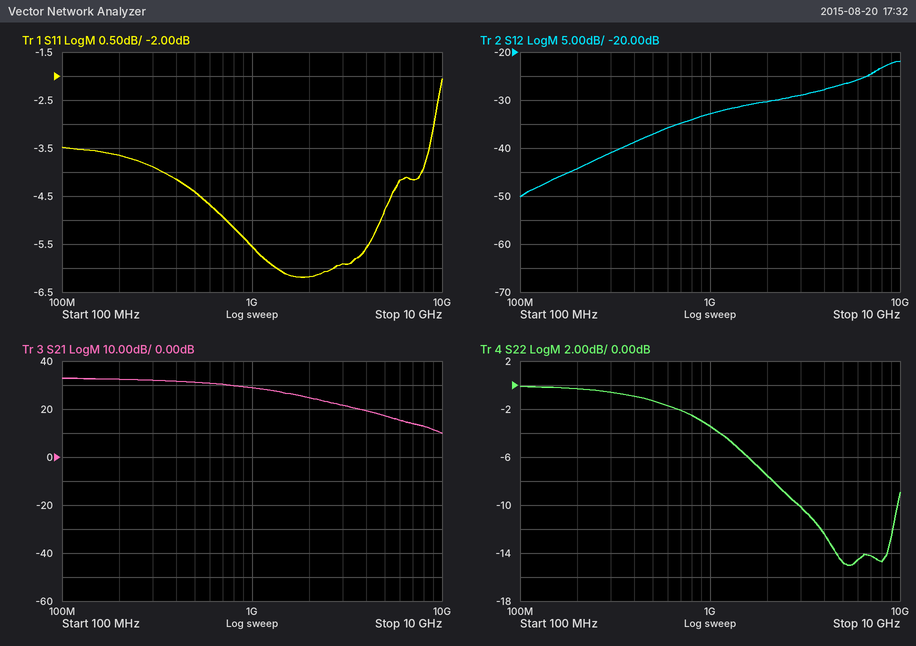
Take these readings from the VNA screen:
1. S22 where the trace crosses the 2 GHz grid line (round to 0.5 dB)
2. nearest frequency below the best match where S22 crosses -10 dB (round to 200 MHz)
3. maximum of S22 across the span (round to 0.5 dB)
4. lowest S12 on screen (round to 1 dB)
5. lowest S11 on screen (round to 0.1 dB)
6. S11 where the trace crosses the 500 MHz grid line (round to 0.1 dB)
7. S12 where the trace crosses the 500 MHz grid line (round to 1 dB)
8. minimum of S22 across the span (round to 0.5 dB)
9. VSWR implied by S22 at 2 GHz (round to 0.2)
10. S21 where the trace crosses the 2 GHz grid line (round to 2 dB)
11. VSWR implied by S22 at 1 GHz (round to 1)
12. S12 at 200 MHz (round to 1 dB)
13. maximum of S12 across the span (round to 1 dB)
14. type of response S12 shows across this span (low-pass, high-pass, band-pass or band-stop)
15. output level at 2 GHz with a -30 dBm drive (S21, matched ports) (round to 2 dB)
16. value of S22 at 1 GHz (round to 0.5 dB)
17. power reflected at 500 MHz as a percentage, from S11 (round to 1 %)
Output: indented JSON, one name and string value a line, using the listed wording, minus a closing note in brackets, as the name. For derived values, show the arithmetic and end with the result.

{
  "S22 where the trace crosses the 2 GHz grid line": "-7.5 dB",
  "nearest frequency below the best match where S22 crosses -10 dB": "3.0 GHz",
  "maximum of S22 across the span": "0.0 dB",
  "lowest S12 on screen": "-50 dB",
  "lowest S11 on screen": "-6.2 dB",
  "S11 where the trace crosses the 500 MHz grid line": "-4.4 dB",
  "S12 where the trace crosses the 500 MHz grid line": "-37 dB",
  "minimum of S22 across the span": "-15.0 dB",
  "VSWR implied by S22 at 2 GHz": "|Γ| = 10^(-7.5/20) = 0.4217; VSWR = (1 + 0.4217)/(1 − 0.4217) ≈ 2.46, so 2.4 to the nearest 0.2",
  "S21 where the trace crosses the 2 GHz grid line": "24 dB",
  "VSWR implied by S22 at 1 GHz": "|Γ| = 10^(-3.5/20) = 0.6683; VSWR = (1 + 0.6683)/(1 − 0.6683) ≈ 5",
  "S12 at 200 MHz": "-44 dB",
  "maximum of S12 across the span": "-22 dB",
  "type of response S12 shows across this span": "high-pass",
  "output level at 2 GHz with a -30 dBm drive (S21, matched ports)": "-30 dBm + (24 dB) = -6 dBm",
  "value of S22 at 1 GHz": "-3.5 dB",
  "power reflected at 500 MHz as a percentage, from S11": "10^(-4.4/10) ≈ 36 %"
}
